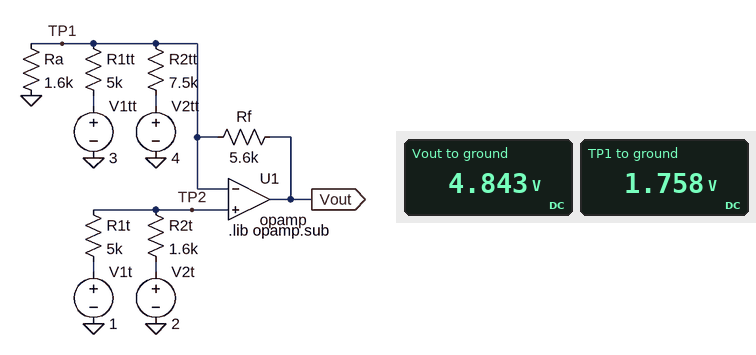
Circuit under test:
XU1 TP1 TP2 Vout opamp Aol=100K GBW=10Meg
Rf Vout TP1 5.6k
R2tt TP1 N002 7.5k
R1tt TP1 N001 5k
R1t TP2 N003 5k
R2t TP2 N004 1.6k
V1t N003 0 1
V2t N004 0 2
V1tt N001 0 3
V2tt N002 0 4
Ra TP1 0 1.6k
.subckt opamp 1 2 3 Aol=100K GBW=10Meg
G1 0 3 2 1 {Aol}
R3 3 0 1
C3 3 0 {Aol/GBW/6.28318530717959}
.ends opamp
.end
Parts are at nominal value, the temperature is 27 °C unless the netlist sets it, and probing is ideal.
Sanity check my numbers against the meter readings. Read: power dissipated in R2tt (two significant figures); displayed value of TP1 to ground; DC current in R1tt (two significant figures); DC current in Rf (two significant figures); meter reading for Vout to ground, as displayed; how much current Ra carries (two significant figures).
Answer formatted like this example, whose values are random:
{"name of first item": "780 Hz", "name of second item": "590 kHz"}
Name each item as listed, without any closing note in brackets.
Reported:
{"power dissipated in R2tt": "670 µW", "displayed value of TP1 to ground": "1.758 V", "DC current in R1tt": "250 µA", "DC current in Rf": "550 µA", "meter reading for Vout to ground, as displayed": "4.843 V", "how much current Ra carries": "1.1 mA"}
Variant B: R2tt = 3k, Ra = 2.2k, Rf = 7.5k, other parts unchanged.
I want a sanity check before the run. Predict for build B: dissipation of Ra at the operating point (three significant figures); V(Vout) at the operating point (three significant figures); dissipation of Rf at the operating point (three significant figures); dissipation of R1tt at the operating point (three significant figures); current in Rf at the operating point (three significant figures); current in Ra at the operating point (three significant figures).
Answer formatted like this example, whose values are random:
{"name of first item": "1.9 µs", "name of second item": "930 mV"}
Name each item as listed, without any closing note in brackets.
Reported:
{"dissipation of Ra at the operating point": "1.40 mW", "V(Vout) at the operating point": "280 mV", "dissipation of Rf at the operating point": "291 µW", "dissipation of R1tt at the operating point": "309 µW", "current in Rf at the operating point": "197 µA", "current in Ra at the operating point": "799 µA"}
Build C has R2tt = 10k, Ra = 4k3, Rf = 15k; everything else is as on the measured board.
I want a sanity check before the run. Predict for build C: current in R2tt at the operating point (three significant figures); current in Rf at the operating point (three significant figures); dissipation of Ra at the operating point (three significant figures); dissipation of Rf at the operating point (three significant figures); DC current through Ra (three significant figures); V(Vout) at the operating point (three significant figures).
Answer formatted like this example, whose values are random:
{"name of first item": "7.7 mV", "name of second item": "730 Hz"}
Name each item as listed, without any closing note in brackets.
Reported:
{"current in R2tt at the operating point": "224 µA", "current in Rf at the operating point": "64.0 µA", "dissipation of Ra at the operating point": "718 µW", "dissipation of Rf at the operating point": "61.4 µW", "DC current through Ra": "409 µA", "V(Vout) at the operating point": "798 mV"}
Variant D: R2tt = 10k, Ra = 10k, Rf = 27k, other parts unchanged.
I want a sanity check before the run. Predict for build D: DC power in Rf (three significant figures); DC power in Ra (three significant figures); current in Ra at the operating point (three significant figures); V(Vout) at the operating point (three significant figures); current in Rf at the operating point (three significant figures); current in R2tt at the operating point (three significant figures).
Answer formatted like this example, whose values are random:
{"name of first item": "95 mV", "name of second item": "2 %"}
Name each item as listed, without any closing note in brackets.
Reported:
{"DC power in Rf": "2.38 mW", "DC power in Ra": "309 µW", "current in Ra at the operating point": "176 µA", "V(Vout) at the operating point": "-6.26 V", "current in Rf at the operating point": "297 µA", "current in R2tt at the operating point": "224 µA"}
